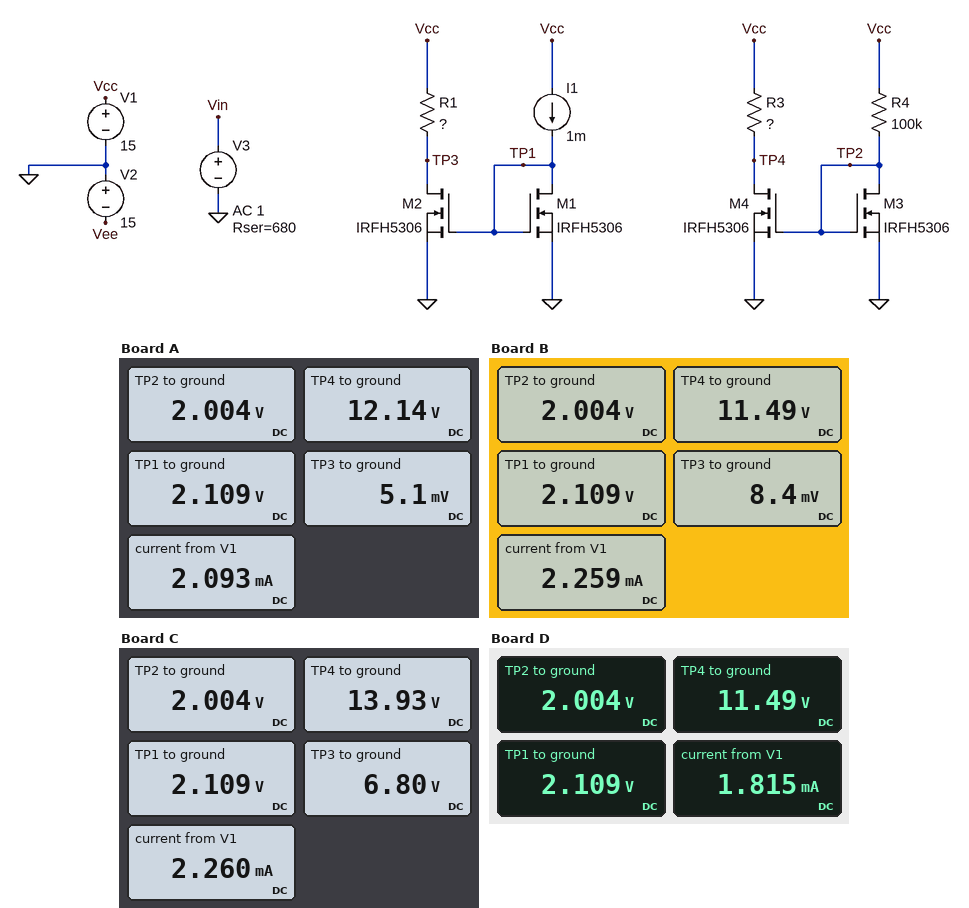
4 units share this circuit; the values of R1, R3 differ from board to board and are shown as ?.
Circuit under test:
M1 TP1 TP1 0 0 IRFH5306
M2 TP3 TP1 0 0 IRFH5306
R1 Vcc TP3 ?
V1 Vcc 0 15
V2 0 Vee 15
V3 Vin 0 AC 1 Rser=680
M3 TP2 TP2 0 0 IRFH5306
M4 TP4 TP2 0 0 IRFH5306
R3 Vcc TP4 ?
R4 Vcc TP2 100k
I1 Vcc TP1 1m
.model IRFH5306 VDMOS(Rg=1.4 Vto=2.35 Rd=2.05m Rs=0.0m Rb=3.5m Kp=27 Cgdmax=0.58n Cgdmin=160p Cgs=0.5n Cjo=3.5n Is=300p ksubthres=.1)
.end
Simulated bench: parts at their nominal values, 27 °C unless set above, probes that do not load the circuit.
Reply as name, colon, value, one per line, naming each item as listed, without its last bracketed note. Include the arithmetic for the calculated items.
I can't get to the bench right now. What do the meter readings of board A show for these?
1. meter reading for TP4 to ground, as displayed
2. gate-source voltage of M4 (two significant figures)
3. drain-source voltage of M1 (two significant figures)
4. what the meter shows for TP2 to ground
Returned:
meter reading for TP4 to ground, as displayed: 12.14 V
gate-source voltage of M4: 2.004 V = 2.0 V
drain-source voltage of M1: 2.109 V = 2.1 V
what the meter shows for TP2 to ground: 2.004 V
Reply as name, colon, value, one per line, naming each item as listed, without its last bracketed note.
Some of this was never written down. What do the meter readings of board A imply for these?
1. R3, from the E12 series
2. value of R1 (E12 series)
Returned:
R3, from the E12 series: 22 kΩ
value of R1: 18 kΩ
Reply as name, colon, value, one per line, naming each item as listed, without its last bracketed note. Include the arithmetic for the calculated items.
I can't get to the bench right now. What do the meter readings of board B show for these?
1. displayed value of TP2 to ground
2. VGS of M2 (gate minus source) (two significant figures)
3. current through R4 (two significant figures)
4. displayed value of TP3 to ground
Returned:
displayed value of TP2 to ground: 2.004 V
VGS of M2 (gate minus source): 2.109 V = 2.1 V
current through R4: (15 V - 2.004 V) / 100 kΩ = 130 µA
displayed value of TP3 to ground: 8.4 mV
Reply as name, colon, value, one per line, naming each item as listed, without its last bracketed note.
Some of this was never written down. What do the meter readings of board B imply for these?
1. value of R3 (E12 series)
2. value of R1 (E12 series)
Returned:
value of R3: 27 kΩ
value of R1: 15 kΩ
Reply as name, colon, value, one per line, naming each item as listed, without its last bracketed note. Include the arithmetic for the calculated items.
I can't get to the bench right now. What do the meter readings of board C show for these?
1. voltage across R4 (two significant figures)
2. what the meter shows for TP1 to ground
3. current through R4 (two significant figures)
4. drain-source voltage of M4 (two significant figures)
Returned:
voltage across R4: 15 V - 2.004 V = 13 V
what the meter shows for TP1 to ground: 2.109 V
current through R4: (15 V - 2.004 V) / 100 kΩ = 130 µA
drain-source voltage of M4: 13.93 V = 14 V
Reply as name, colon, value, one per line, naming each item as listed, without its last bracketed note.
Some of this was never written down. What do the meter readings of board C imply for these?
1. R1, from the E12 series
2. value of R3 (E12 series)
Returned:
R1, from the E12 series: 8.2 kΩ
value of R3: 8.2 kΩ
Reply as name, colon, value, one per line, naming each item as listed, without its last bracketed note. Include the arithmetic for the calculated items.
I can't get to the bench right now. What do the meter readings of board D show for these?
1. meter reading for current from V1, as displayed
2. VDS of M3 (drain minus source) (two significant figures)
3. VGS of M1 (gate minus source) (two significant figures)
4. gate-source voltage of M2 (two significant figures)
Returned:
meter reading for current from V1, as displayed: 1.815 mA
VDS of M3 (drain minus source): 2.004 V = 2.0 V
VGS of M1 (gate minus source): 2.109 V = 2.1 V
gate-source voltage of M2: 2.109 V = 2.1 V
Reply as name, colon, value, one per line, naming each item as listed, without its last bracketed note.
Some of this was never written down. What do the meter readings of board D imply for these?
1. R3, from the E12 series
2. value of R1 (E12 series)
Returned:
R3, from the E12 series: 27 kΩ
value of R1: 27 kΩ
